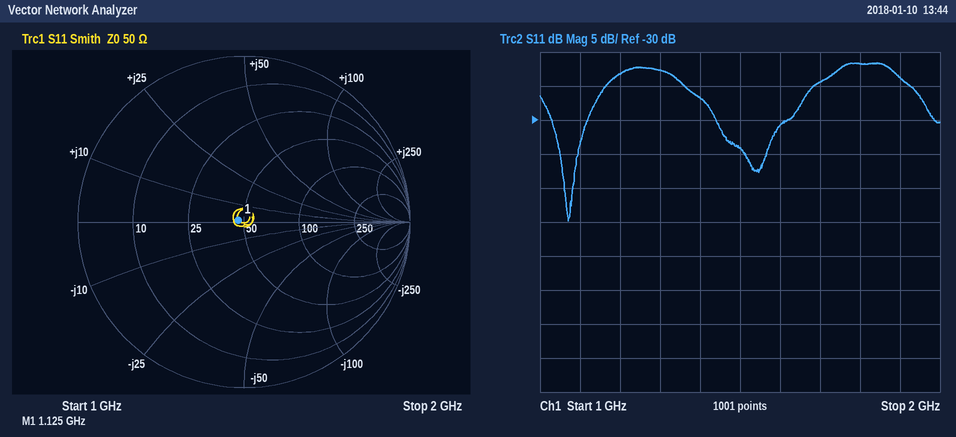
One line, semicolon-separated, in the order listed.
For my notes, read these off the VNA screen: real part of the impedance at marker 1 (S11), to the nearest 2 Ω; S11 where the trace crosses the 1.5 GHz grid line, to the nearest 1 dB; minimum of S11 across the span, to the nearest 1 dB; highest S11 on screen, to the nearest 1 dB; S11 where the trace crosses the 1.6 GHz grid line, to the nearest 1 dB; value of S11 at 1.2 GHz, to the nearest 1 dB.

46 Ω; -34 dB; -45 dB; -22 dB; -31 dB; -23 dB
